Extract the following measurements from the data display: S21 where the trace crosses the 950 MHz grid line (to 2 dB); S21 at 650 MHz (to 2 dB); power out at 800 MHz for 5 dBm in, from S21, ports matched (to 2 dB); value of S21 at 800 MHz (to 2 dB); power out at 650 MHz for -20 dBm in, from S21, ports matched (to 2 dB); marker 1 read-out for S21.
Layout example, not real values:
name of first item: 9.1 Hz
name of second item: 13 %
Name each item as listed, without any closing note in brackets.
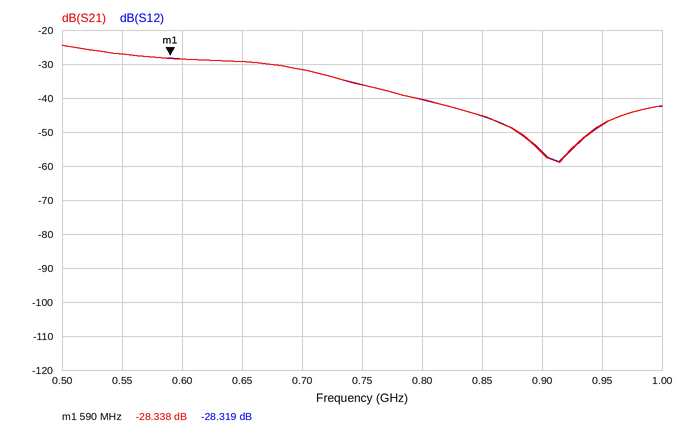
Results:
S21 where the trace crosses the 950 MHz grid line: -48 dB
S21 at 650 MHz: -30 dB
power out at 800 MHz for 5 dBm in, from S21, ports matched: -36 dBm
value of S21 at 800 MHz: -40 dB
power out at 650 MHz for -20 dBm in, from S21, ports matched: -50 dBm
marker 1 read-out for S21: -28.338 dB
